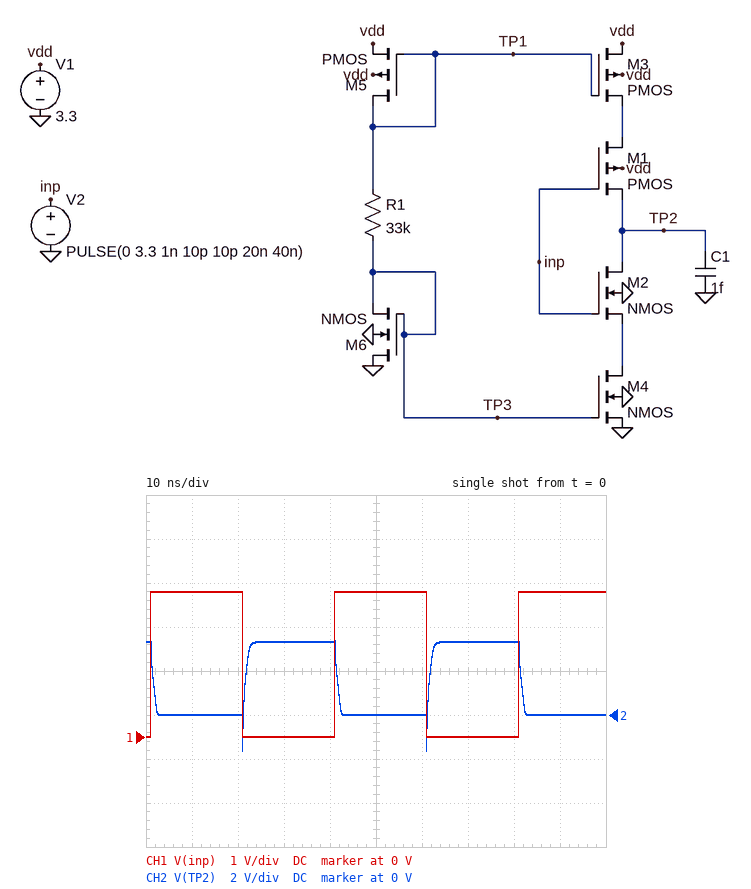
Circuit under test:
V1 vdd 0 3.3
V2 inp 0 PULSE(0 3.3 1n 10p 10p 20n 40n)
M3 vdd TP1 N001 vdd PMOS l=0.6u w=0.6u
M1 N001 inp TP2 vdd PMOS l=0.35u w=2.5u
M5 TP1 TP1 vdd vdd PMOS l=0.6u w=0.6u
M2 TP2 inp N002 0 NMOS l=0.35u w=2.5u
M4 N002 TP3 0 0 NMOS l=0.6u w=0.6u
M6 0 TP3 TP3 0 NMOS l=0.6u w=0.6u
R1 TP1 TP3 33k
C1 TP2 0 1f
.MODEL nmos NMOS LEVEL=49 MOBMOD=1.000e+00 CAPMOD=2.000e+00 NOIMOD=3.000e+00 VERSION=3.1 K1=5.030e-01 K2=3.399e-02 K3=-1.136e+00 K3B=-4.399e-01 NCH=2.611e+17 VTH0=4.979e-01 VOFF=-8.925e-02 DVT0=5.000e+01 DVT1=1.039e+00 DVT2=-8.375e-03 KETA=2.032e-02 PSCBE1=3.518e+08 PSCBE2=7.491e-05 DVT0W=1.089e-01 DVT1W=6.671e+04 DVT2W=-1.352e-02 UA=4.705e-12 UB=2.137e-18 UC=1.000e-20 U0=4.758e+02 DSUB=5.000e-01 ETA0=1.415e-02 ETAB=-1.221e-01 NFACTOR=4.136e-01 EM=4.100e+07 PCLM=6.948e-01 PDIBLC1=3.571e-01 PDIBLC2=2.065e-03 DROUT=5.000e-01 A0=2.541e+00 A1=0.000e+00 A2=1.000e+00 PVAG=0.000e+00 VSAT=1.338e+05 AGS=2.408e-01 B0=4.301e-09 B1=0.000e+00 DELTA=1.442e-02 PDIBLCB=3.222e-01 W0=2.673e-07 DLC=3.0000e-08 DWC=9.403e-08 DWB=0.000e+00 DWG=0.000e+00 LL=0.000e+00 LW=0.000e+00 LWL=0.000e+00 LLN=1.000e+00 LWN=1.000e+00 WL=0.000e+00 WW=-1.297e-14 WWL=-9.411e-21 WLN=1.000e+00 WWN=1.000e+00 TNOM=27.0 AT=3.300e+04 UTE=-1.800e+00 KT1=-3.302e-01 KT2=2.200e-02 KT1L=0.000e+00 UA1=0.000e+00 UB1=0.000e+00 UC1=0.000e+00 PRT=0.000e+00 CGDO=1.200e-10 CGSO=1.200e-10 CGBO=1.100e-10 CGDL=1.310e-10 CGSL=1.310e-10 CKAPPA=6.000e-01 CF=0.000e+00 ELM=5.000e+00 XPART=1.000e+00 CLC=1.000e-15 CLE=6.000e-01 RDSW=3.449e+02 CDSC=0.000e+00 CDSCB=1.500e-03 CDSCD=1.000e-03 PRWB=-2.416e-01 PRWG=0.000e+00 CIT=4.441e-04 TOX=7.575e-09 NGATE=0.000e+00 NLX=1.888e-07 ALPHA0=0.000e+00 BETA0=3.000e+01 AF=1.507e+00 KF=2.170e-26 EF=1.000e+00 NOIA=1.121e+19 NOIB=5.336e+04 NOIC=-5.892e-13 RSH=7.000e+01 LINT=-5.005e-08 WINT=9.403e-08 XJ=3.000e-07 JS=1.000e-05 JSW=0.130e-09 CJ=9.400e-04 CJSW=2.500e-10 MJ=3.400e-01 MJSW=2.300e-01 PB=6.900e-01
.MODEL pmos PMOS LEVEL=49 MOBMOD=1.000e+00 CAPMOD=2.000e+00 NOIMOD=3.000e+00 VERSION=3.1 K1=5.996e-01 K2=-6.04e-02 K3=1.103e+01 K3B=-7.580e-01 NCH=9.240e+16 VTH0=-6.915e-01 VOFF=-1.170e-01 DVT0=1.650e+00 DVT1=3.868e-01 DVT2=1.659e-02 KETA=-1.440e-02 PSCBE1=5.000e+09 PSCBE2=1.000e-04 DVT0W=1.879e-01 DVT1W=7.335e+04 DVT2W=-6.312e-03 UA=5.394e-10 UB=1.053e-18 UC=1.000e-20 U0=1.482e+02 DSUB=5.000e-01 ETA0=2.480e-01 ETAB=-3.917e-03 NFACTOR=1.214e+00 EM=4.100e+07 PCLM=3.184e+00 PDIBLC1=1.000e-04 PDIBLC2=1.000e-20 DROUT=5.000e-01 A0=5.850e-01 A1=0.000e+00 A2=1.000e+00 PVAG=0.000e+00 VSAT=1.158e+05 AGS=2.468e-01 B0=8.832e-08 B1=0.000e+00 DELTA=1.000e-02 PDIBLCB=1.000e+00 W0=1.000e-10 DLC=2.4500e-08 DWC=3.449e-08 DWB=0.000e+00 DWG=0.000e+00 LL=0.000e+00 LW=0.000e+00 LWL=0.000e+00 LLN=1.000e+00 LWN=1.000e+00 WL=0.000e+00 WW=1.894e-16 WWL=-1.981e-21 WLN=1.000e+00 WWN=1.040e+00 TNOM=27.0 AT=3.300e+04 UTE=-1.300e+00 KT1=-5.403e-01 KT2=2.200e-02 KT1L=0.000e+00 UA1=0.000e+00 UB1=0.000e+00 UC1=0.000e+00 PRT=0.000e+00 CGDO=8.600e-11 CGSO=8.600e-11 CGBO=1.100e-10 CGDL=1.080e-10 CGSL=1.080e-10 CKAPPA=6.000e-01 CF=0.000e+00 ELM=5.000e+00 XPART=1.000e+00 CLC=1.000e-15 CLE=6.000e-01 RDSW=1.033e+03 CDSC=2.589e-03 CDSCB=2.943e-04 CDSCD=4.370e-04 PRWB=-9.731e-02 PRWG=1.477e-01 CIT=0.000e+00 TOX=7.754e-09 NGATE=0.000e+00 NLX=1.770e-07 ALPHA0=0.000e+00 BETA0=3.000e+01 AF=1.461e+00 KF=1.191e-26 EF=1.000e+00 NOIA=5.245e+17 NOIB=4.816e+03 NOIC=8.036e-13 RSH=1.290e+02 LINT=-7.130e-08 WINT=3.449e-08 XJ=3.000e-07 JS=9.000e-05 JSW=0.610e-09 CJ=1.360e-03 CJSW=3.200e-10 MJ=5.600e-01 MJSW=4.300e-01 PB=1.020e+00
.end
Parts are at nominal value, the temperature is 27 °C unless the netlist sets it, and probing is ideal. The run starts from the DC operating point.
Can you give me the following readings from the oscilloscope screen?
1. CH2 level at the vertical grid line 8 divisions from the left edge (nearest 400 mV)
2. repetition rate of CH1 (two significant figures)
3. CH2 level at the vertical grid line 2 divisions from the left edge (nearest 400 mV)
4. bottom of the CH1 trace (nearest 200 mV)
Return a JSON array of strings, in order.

["3.2 V", "25 MHz", "0 V", "0 V"]
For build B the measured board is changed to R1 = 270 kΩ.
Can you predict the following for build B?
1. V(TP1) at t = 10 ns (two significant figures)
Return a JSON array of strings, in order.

["2.0 V"]
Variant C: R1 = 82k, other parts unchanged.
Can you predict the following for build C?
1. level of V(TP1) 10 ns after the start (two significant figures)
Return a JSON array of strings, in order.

["1.8 V"]
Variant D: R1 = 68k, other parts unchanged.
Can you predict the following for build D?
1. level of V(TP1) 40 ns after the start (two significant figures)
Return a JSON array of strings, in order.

["1.7 V"]
